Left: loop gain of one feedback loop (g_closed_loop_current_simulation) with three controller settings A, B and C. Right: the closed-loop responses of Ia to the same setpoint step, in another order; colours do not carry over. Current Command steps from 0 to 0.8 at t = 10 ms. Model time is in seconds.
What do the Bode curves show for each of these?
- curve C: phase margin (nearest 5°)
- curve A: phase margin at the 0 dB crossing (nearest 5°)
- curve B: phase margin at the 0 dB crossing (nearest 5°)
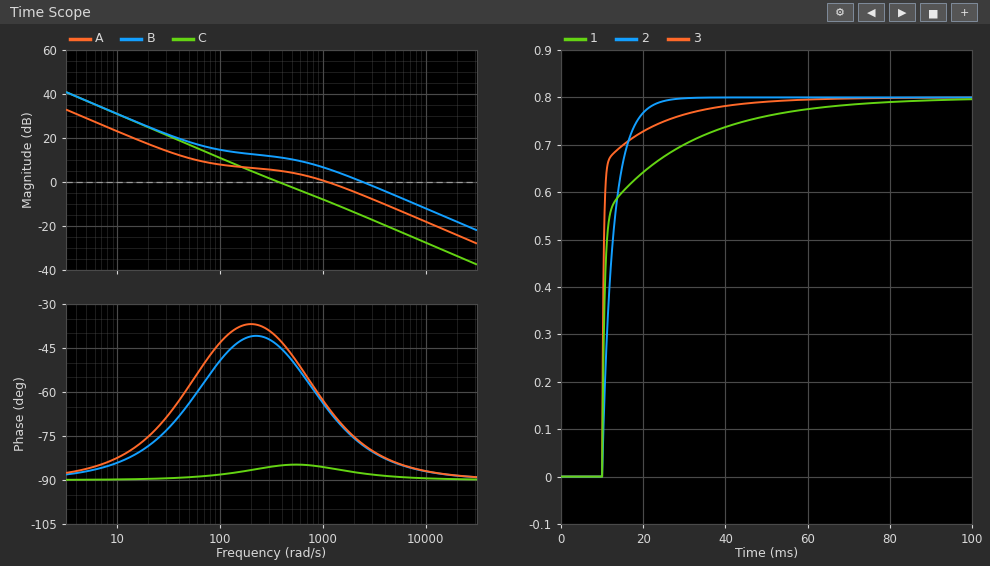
95°
115°
100°
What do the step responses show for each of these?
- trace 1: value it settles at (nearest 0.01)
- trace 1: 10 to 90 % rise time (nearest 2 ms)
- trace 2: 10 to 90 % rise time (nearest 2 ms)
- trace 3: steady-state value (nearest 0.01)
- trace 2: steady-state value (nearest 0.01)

0.80
24 ms
6 ms
0.80
0.80
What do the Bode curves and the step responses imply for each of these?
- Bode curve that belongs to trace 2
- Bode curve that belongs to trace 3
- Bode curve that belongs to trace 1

C
B
A
